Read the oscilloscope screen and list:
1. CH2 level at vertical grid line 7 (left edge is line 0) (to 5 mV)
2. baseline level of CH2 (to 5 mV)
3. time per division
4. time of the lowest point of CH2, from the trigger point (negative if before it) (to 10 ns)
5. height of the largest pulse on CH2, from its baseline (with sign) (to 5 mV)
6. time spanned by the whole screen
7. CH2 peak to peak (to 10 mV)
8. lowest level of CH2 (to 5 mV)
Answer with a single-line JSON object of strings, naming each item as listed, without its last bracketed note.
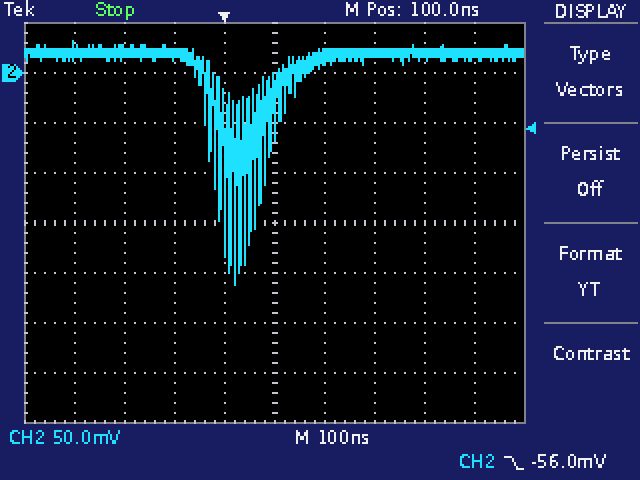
{"CH2 level at vertical grid line 7 (left edge is line 0)": "20 mV", "baseline level of CH2": "20 mV", "time per division": "100 ns", "time of the lowest point of CH2, from the trigger point (negative if before it)": "+20 ns", "height of the largest pulse on CH2, from its baseline (with sign)": "-230 mV", "time spanned by the whole screen": "1 µs", "CH2 peak to peak": "240 mV", "lowest level of CH2": "-210 mV"}
